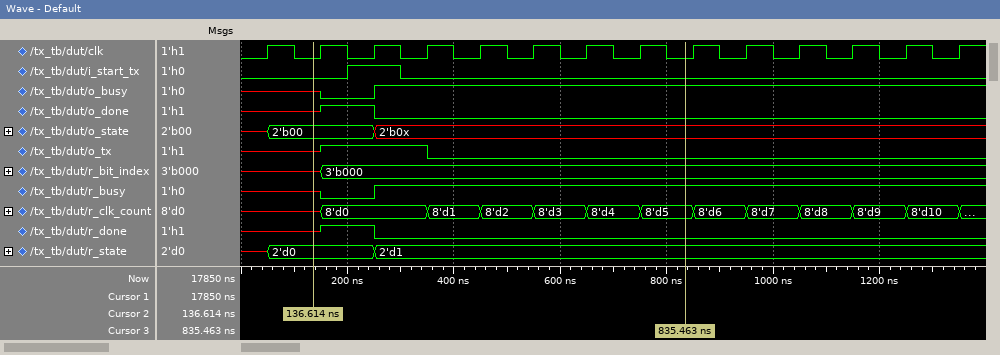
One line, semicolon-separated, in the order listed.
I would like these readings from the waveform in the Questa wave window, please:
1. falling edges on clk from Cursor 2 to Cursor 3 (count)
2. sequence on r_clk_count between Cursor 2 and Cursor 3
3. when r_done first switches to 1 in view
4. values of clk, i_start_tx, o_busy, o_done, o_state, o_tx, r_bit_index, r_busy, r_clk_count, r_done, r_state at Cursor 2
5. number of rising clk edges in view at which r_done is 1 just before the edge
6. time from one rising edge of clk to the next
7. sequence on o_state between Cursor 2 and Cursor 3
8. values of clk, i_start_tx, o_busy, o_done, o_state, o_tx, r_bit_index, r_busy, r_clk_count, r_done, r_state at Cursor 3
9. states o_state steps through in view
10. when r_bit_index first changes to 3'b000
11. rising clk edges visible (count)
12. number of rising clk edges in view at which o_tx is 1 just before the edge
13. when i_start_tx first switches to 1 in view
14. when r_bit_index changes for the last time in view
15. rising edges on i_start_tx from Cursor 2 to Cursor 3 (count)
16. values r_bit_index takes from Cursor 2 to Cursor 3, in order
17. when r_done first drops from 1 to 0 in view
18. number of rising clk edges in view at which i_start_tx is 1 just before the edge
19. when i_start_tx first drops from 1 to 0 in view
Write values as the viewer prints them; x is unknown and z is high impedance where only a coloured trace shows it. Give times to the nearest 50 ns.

7; x, 8'd0, 8'd1, 8'd2, 8'd3, 8'd4, 8'd5; 150 ns; clk=0, i_start_tx=0, o_busy=x, o_done=x, o_state=2'b00, o_tx=x, r_bit_index=x, r_busy=x, r_clk_count=x, r_done=x, r_state=2'd0; 1; 100 ns; 2'b00, 2'b0x; clk=0, i_start_tx=0, o_busy=1, o_done=0, o_state=2'b0x, o_tx=0, r_bit_index=3'b000, r_busy=1, r_clk_count=8'd5, r_done=0, r_state=2'd1; x, 2'b00, 2'b0x; 150 ns; 14; 2; 200 ns; 150 ns; 1; x, 3'b000; 250 ns; 1; 300 ns
